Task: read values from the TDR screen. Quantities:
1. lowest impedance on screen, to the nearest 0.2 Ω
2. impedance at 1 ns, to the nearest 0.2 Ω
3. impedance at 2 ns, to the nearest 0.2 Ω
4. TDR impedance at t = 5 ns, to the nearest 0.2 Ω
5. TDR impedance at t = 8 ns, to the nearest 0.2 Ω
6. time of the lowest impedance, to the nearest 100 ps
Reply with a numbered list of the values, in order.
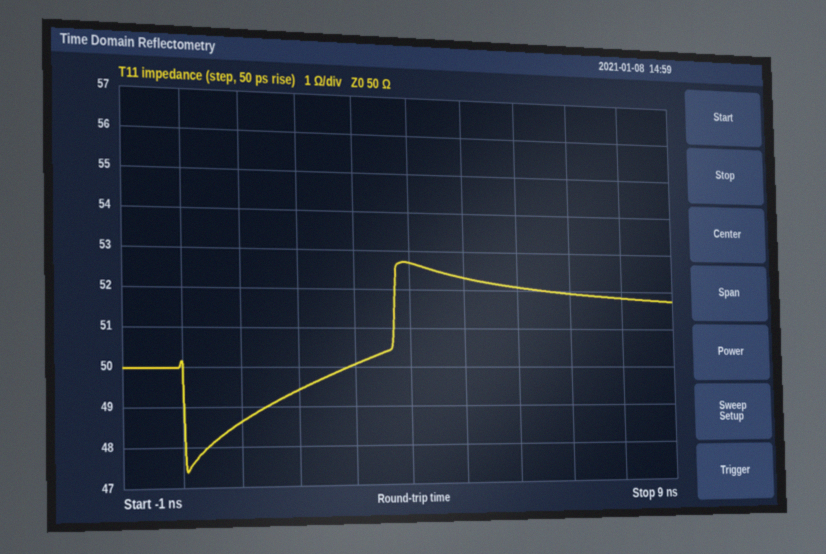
1. 47.4 Ω
2. 48.6 Ω
3. 49.4 Ω
4. 52.4 Ω
5. 51.8 Ω
6. 100 ps
